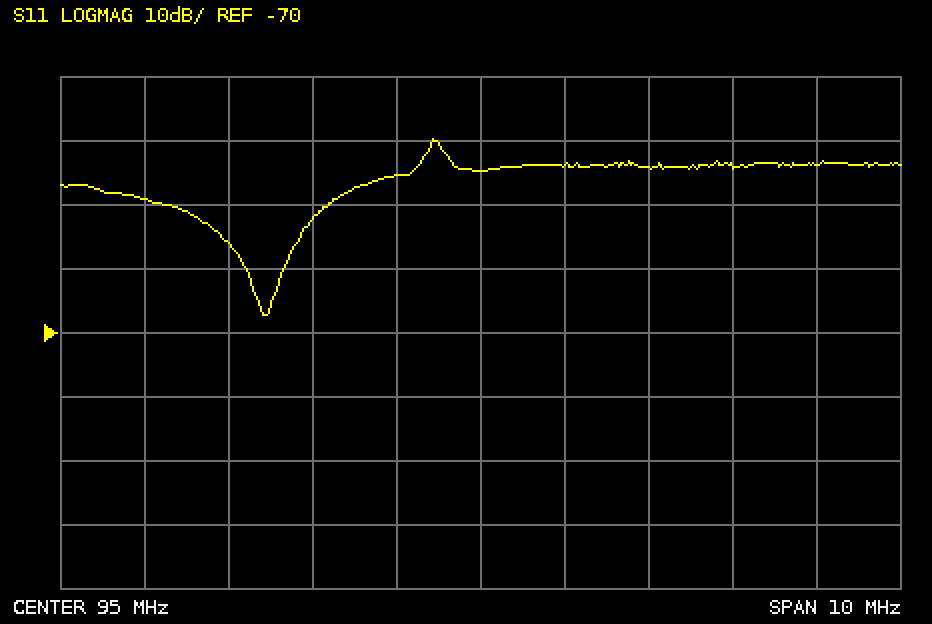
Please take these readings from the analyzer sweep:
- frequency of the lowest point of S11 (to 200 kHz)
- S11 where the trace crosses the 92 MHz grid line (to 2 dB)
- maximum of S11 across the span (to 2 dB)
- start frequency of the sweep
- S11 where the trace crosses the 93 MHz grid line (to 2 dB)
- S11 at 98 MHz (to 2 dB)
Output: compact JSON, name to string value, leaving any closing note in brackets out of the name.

{"frequency of the lowest point of S11": "92.4 MHz", "S11 where the trace crosses the 92 MHz grid line": "-56 dB", "maximum of S11 across the span": "-40 dB", "start frequency of the sweep": "90 MHz", "S11 where the trace crosses the 93 MHz grid line": "-52 dB", "S11 at 98 MHz": "-44 dB"}
